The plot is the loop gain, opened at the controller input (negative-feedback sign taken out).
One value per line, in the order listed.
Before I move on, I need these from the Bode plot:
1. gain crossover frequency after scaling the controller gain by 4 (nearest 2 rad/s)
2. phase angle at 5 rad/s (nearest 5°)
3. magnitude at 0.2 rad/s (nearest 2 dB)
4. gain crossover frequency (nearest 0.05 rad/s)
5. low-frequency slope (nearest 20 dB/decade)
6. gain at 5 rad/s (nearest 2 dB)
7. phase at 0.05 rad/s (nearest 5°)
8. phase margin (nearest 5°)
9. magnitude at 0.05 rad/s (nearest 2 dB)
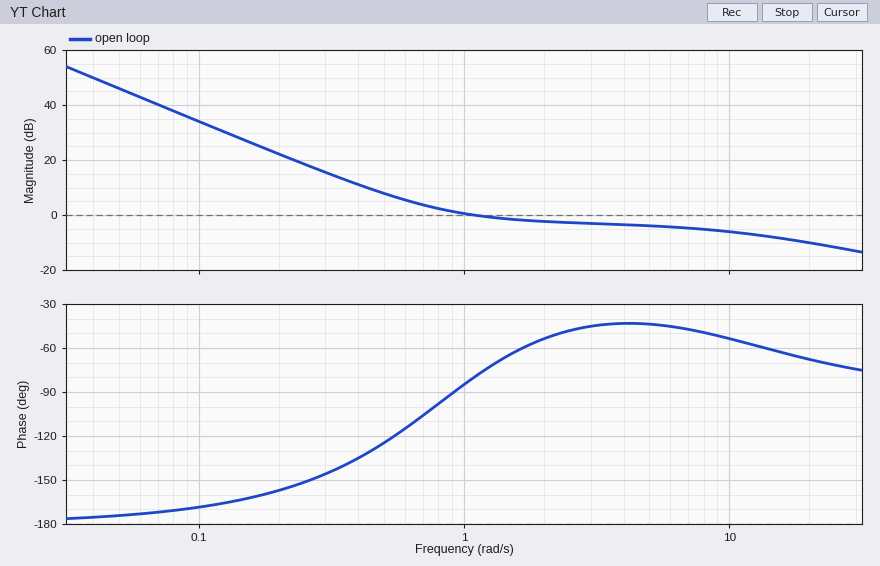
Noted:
26 rad/s
-45°
22 dB
1.10 rad/s
-40 dB/decade
-4 dB
-175°
100°
46 dB
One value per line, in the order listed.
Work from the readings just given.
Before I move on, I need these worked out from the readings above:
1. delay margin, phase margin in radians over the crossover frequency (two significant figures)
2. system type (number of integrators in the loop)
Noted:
1.6 s
2
